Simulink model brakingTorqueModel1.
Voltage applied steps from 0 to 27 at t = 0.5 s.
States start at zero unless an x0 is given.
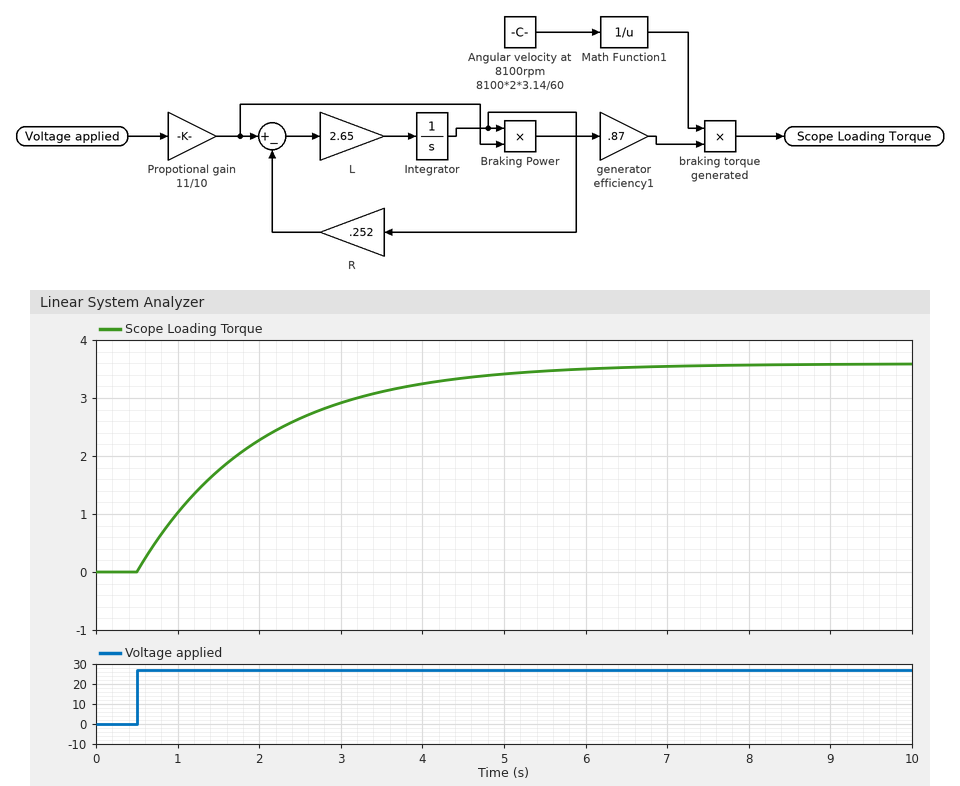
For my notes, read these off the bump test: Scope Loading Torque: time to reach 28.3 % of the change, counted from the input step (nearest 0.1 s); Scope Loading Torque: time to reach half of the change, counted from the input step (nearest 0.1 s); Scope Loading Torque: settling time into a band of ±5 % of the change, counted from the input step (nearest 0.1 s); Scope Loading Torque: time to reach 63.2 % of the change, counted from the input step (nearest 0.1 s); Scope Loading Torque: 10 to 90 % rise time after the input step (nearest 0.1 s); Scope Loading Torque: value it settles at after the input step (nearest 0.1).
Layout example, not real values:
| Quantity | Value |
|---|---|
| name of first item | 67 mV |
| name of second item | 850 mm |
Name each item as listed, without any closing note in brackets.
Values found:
| Quantity | Value |
|---|---|
| Scope Loading Torque: time to reach 28.3 % of the change, counted from the input step | 0.5 s |
| Scope Loading Torque: time to reach half of the change, counted from the input step | 1.0 s |
| Scope Loading Torque: settling time into a band of ±5 % of the change, counted from the input step | 4.5 s |
| Scope Loading Torque: time to reach 63.2 % of the change, counted from the input step | 1.5 s |
| Scope Loading Torque: 10 to 90 % rise time after the input step | 3.3 s |
| Scope Loading Torque: value it settles at after the input step | 3.6 |
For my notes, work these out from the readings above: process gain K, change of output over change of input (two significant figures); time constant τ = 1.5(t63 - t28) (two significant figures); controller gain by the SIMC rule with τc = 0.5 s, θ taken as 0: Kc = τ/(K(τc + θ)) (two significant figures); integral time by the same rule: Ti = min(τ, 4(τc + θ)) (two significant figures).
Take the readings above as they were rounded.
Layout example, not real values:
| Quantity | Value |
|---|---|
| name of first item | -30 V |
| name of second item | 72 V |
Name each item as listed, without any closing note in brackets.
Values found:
| Quantity | Value |
|---|---|
| process gain K, change of output over change of input | 0.13 |
| time constant τ = 1.5(t63 - t28) | 1.5 s |
| controller gain by the SIMC rule with τc = 0.5 s, θ taken as 0: Kc = τ/(K(τc + θ)) | 23 |
| integral time by the same rule: Ti = min(τ, 4(τc + θ)) | 1.5 s |
